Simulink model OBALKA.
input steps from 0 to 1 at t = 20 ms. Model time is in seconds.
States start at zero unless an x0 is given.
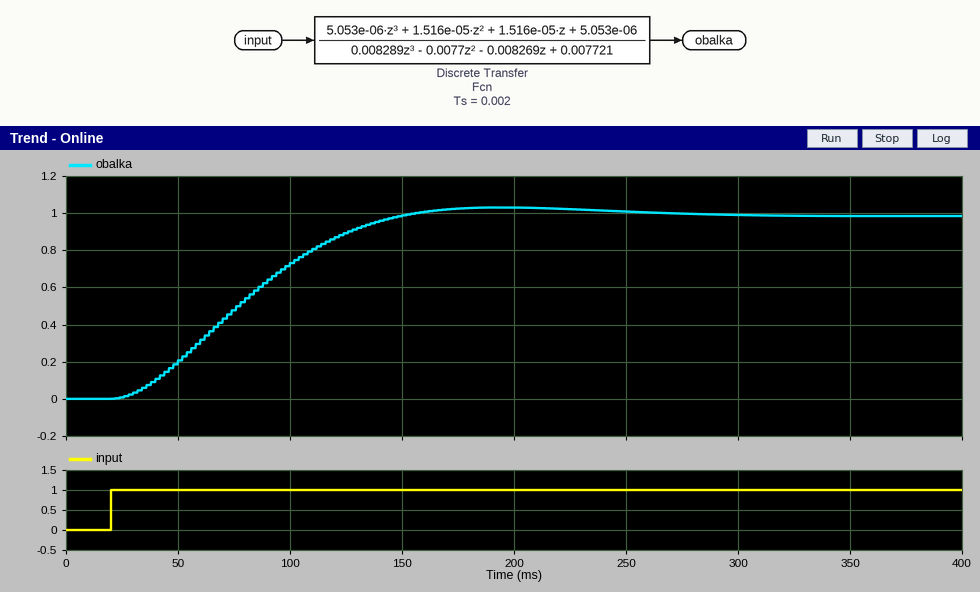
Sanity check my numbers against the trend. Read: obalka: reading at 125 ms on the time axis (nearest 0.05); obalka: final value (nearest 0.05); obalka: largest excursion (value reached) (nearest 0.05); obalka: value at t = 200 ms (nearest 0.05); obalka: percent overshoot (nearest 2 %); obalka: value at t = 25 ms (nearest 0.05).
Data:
0.90
1.00
1.05
1.05
4 %
0.00
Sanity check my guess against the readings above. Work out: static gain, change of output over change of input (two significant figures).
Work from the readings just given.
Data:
1.0
